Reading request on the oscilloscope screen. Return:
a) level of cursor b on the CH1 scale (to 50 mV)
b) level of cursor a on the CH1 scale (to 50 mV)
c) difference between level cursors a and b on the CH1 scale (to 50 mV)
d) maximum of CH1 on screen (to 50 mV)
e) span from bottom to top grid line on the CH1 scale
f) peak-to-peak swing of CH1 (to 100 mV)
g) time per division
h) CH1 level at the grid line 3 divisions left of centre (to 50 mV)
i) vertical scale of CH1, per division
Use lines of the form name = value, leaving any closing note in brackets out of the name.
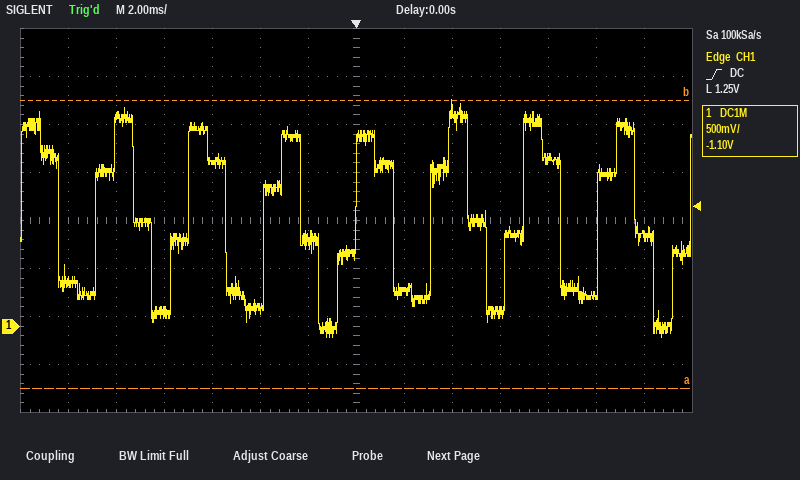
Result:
level of cursor b on the CH1 scale = 2.35 V
level of cursor a on the CH1 scale = -650 mV
difference between level cursors a and b on the CH1 scale = 3.00 V
maximum of CH1 on screen = 2.35 V
span from bottom to top grid line on the CH1 scale = 4 V
peak-to-peak swing of CH1 = 2.50 V
time per division = 2 ms
CH1 level at the grid line 3 divisions left of centre = 1.70 V
vertical scale of CH1, per division = 500 mV
